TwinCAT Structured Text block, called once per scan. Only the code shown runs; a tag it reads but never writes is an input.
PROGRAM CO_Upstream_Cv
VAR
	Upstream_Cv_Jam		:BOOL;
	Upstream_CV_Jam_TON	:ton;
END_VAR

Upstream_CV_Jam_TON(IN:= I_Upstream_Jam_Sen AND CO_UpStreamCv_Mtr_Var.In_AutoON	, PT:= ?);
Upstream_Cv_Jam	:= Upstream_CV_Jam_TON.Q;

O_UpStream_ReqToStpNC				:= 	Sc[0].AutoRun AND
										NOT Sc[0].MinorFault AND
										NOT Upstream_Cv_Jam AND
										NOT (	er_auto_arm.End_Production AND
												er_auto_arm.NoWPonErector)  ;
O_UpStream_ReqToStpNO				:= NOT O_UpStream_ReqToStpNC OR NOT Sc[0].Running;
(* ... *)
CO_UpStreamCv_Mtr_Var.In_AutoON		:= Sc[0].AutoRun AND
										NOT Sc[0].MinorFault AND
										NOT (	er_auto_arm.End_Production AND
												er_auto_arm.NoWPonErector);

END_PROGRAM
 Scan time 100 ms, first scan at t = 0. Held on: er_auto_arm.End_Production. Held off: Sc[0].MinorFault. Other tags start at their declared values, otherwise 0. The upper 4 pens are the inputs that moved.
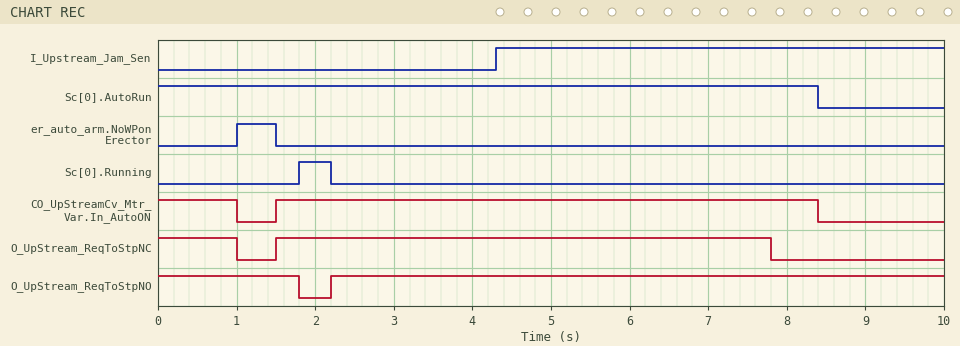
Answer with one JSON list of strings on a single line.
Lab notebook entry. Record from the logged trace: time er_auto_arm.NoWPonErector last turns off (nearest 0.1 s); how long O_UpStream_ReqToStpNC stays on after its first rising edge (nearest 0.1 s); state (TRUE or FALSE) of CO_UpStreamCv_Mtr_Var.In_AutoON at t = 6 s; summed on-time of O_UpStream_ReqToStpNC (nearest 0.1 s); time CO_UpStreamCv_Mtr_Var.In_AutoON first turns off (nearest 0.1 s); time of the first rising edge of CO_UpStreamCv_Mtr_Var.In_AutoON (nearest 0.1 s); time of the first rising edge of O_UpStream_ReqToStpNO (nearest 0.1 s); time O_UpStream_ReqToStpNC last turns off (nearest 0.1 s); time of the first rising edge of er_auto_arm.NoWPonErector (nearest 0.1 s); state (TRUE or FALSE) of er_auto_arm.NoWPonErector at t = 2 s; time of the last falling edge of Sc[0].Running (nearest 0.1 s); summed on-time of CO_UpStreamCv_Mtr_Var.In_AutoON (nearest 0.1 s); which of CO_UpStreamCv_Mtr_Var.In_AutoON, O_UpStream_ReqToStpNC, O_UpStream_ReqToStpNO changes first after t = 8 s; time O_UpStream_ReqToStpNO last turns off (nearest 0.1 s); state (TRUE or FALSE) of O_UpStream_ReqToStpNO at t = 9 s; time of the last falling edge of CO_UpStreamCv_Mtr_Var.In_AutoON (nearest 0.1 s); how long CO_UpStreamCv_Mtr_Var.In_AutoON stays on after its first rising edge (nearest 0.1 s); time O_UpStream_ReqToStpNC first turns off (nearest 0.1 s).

["1.5 s", "6.3 s", "TRUE", "7.3 s", "1.0 s", "1.5 s", "2.2 s", "7.8 s", "1.0 s", "FALSE", "2.2 s", "7.9 s", "CO_UpStreamCv_Mtr_Var.In_AutoON", "1.8 s", "TRUE", "8.4 s", "6.9 s", "1.0 s"]
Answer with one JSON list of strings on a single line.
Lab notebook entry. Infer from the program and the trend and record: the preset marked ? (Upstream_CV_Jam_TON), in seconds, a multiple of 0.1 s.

["3.5 s"]
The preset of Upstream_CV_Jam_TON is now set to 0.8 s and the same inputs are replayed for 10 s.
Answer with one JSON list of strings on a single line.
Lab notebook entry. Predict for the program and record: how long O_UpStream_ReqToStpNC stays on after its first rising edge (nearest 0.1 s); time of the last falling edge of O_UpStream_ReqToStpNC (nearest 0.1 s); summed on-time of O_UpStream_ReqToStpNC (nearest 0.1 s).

["3.6 s", "5.1 s", "4.6 s"]
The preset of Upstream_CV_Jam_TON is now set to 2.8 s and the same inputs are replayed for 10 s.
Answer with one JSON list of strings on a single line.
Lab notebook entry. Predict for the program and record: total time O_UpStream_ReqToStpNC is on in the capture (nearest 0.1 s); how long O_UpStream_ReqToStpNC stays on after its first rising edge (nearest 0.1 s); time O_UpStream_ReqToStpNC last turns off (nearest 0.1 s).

["6.6 s", "5.6 s", "7.1 s"]
